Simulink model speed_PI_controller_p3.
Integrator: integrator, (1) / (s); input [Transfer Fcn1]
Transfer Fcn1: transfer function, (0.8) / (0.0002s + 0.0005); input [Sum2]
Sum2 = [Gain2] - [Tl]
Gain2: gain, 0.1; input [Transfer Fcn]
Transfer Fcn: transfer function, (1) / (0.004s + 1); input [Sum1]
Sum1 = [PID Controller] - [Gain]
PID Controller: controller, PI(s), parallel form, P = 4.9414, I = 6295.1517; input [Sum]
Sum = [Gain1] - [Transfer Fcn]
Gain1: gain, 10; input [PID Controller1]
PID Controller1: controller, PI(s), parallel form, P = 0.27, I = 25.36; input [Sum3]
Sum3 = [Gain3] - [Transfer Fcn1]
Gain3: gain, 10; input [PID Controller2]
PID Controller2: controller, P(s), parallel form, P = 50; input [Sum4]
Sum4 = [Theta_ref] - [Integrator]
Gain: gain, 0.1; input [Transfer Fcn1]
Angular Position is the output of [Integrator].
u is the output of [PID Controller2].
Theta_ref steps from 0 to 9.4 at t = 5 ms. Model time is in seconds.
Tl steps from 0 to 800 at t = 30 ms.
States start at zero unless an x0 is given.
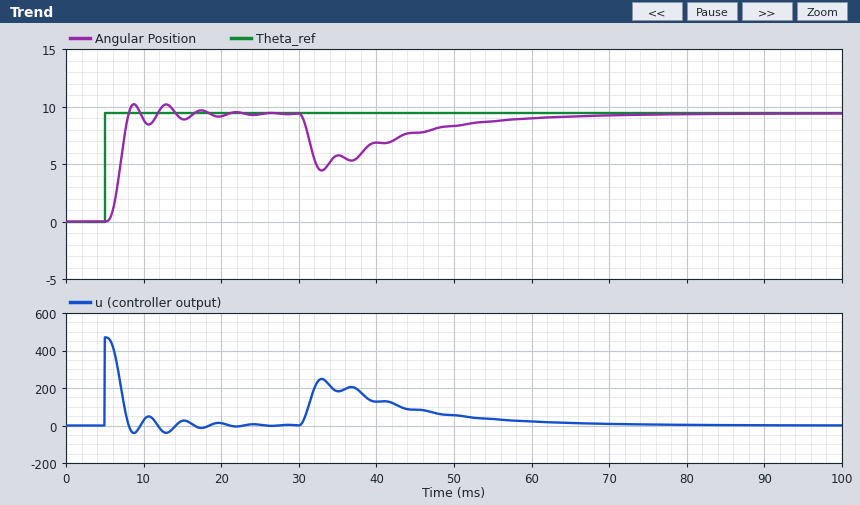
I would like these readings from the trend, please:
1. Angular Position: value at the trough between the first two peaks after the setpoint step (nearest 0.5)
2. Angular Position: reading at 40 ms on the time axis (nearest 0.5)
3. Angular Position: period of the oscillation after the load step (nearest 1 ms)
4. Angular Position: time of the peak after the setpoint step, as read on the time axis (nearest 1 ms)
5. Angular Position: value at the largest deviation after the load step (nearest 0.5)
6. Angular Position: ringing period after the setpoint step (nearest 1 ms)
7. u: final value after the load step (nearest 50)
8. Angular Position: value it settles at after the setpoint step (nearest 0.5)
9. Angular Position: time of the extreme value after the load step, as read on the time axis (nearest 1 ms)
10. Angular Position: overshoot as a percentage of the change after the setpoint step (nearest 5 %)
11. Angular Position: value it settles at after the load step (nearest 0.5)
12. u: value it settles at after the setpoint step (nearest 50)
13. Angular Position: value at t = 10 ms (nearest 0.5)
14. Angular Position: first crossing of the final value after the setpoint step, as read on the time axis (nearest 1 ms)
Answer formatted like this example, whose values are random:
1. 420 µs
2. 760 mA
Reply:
1. 8.5
2. 7.0
3. 4 ms
4. 9 ms
5. 4.5
6. 4 ms
7. 0
8. 9.5
9. 33 ms
10. 10 %
11. 9.5
12. 0
13. 9.0
14. 8 ms
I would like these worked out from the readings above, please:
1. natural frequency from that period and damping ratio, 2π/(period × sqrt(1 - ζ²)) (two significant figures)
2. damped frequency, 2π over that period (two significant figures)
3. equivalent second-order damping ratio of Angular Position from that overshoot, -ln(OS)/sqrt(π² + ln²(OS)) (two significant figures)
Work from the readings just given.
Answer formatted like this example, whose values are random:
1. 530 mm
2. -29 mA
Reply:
1. 1.9 rad/ms
2. 1.6 rad/ms
3. 0.59
